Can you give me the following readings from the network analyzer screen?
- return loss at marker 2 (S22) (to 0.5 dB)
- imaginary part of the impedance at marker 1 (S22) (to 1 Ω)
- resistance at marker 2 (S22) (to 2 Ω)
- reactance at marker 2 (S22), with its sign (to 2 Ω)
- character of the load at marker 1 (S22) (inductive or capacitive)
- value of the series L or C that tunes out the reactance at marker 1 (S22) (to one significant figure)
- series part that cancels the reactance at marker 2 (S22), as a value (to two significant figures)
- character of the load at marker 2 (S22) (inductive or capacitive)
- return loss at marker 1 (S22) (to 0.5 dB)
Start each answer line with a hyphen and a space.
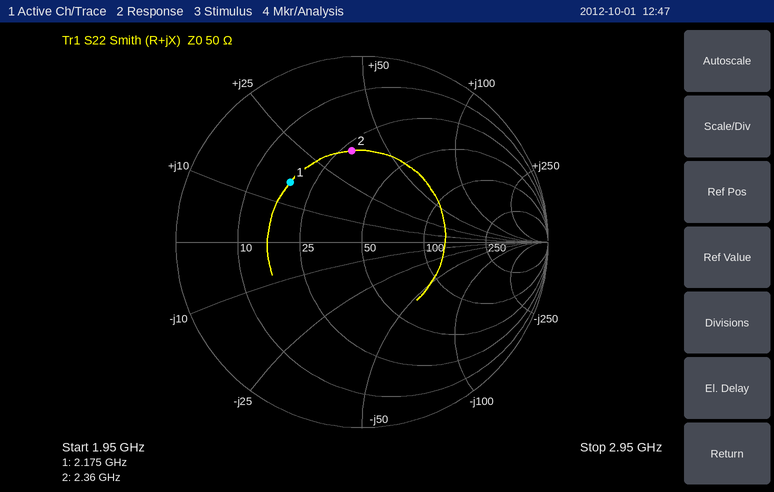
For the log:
- 6.0 dB
- +16 Ω
- 28 Ω
- +36 Ω
- inductive
- 5 pF
- 1.9 pF
- inductive
- 6.0 dB
